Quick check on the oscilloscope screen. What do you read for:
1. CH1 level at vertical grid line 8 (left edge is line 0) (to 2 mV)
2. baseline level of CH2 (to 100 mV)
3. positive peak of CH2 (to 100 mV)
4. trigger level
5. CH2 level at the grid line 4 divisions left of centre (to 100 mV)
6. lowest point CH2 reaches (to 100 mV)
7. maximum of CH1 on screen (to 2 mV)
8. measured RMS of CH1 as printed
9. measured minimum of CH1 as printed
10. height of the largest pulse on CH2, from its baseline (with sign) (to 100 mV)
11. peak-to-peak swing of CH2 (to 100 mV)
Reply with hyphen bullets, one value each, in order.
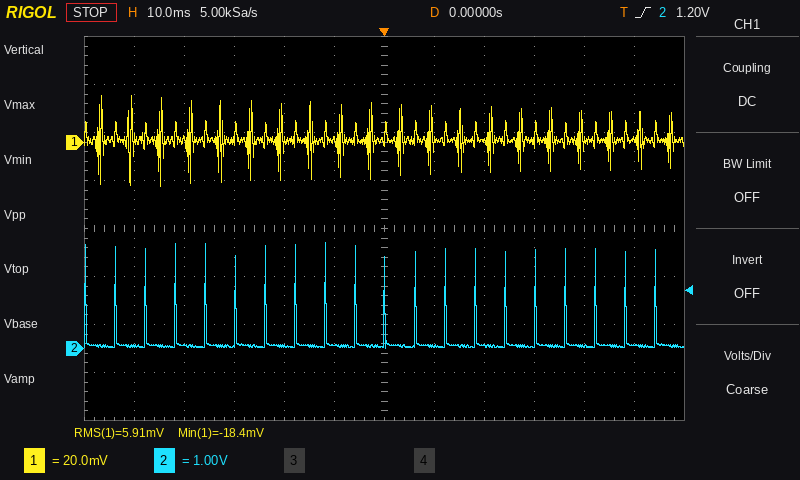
- 0 mV
- 100 mV
- 2.2 V
- 1.20 V
- 100 mV
- 0.0 V
- 20 mV
- 5.91 mV
- -18.4 mV
- +2.1 V
- 2.2 V
